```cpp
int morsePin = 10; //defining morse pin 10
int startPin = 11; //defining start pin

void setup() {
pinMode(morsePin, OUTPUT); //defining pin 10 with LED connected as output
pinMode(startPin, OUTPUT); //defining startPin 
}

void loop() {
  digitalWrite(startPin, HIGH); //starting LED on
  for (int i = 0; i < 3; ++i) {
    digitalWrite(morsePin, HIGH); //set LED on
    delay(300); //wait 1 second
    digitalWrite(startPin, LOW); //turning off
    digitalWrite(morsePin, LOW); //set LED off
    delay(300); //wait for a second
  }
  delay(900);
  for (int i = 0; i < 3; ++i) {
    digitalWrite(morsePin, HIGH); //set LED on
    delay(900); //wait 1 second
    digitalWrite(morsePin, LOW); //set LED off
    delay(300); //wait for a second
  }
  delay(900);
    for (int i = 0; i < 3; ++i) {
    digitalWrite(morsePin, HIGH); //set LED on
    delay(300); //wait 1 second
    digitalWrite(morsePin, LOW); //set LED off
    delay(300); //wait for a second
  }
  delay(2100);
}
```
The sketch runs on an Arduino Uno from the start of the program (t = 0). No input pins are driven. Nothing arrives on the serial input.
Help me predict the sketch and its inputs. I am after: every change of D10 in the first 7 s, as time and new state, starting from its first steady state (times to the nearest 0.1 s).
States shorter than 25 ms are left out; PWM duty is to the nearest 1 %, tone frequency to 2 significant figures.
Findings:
0 s high; 0.3 s low; 0.6 s high; 0.9 s low; 1.2 s high; 1.5 s low; 2.7 s high; 3.6 s low; 3.9 s high; 4.8 s low; 5.1 s high; 6 s low
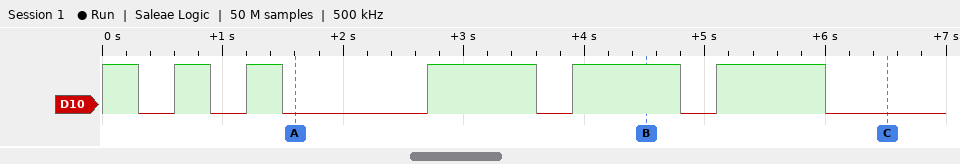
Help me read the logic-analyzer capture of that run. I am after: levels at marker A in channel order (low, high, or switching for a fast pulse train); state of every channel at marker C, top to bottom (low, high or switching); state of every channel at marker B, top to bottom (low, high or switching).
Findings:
D10 low
D10 low
D10 high
